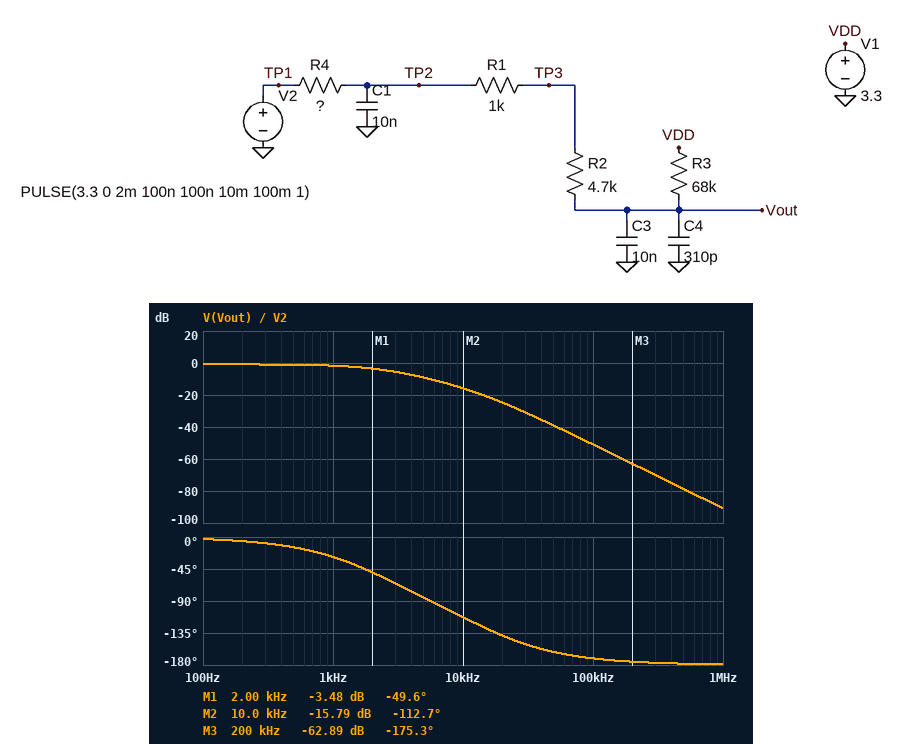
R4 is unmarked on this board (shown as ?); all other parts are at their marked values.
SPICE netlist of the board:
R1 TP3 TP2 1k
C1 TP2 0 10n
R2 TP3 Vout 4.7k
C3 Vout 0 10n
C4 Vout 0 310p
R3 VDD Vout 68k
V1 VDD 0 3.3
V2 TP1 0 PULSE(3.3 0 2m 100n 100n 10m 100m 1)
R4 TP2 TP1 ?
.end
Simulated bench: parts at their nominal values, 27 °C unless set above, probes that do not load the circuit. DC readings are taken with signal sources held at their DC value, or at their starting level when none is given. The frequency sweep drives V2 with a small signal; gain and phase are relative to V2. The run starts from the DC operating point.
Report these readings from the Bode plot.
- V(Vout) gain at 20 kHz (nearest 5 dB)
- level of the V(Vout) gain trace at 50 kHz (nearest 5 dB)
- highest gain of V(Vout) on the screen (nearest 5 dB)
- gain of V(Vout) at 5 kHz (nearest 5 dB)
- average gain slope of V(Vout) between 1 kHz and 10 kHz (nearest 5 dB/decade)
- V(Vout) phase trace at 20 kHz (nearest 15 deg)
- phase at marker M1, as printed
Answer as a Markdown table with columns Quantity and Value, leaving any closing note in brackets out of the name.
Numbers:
| Quantity | Value |
|---|---|
| V(Vout) gain at 20 kHz | -25 dB |
| level of the V(Vout) gain trace at 50 kHz | -40 dB |
| highest gain of V(Vout) on the screen | 0 dB |
| gain of V(Vout) at 5 kHz | -10 dB |
| average gain slope of V(Vout) between 1 kHz and 10 kHz | -15 dB/decade |
| V(Vout) phase trace at 20 kHz | -135 deg |
| phase at marker M1, as printed | -49.6 deg |
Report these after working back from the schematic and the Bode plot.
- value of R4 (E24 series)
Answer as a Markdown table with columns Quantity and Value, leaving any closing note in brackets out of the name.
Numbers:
| Quantity | Value |
|---|---|
| value of R4 | 1.5 kΩ |
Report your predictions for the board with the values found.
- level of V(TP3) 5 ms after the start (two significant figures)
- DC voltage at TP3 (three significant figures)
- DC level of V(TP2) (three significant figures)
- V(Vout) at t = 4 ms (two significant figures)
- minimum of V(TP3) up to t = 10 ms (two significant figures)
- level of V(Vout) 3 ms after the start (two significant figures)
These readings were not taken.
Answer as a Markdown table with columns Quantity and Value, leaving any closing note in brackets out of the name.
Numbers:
| Quantity | Value |
|---|---|
| level of V(TP3) 5 ms after the start | 110 mV |
| DC voltage at TP3 | 3.30 V |
| DC level of V(TP2) | 3.30 V |
| V(Vout) at t = 4 ms | 320 mV |
| minimum of V(TP3) up to t = 10 ms | 110 mV |
| level of V(Vout) 3 ms after the start | 320 mV |
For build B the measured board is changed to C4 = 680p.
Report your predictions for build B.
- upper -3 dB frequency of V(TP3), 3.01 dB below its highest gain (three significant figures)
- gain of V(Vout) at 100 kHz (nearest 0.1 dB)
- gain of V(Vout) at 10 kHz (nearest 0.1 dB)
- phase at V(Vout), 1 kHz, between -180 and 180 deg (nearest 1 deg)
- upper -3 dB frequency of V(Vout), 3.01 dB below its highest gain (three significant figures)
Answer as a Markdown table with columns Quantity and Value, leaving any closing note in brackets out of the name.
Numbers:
| Quantity | Value |
|---|---|
| upper -3 dB frequency of V(TP3), 3.01 dB below its highest gain | 4.12 kHz |
| gain of V(Vout) at 100 kHz | -51.2 dB |
| gain of V(Vout) at 10 kHz | -16.1 dB |
| phase at V(Vout), 1 kHz, between -180 and 180 deg | -29 deg |
| upper -3 dB frequency of V(Vout), 3.01 dB below its highest gain | 2.13 kHz |
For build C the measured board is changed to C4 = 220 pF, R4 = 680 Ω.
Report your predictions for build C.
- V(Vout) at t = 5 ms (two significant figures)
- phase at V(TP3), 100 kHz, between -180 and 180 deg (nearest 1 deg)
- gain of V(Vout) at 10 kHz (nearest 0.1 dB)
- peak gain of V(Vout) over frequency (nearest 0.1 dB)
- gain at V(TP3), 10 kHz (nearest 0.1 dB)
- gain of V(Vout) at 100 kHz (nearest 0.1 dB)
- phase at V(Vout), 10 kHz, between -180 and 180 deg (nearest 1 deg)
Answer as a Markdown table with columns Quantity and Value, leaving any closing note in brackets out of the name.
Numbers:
| Quantity | Value |
|---|---|
| V(Vout) at t = 5 ms | 280 mV |
| phase at V(TP3), 100 kHz, between -180 and 180 deg | -76 deg |
| gain of V(Vout) at 10 kHz | -13.2 dB |
| peak gain of V(Vout) over frequency | -0.8 dB |
| gain at V(TP3), 10 kHz | -3.1 dB |
| gain of V(Vout) at 100 kHz | -44.2 dB |
| phase at V(Vout), 10 kHz, between -180 and 180 deg | -96 deg |
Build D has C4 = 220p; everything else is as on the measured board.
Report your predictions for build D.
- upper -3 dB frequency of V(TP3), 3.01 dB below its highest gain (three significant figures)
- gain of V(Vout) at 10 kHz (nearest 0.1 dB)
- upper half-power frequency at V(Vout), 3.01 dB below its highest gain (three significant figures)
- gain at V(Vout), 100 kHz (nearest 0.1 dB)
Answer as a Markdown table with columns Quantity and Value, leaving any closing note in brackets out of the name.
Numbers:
| Quantity | Value |
|---|---|
| upper -3 dB frequency of V(TP3), 3.01 dB below its highest gain | 4.22 kHz |
| gain of V(Vout) at 10 kHz | -15.7 dB |
| upper half-power frequency at V(Vout), 3.01 dB below its highest gain | 2.22 kHz |
| gain at V(Vout), 100 kHz | -50.8 dB |
